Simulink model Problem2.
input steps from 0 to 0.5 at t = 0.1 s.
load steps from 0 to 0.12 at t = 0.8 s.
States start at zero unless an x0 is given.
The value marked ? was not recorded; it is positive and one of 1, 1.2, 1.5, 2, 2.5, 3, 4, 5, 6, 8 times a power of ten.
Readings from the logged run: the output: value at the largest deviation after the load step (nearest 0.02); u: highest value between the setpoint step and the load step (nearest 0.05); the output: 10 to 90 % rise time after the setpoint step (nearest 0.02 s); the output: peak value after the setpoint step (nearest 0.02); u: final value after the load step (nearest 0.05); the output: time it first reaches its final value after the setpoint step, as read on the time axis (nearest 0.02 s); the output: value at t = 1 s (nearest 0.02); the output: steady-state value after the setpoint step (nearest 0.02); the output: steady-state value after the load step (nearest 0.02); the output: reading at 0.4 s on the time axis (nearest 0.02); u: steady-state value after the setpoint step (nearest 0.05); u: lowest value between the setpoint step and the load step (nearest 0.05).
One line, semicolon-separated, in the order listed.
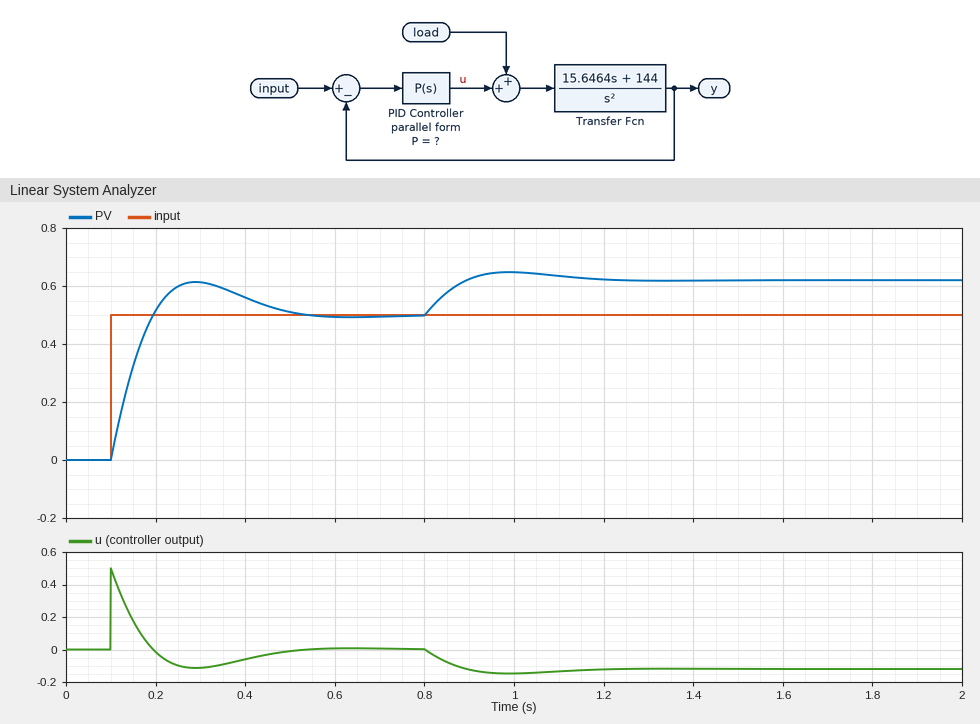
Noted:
0.64; 0.50; 0.08 s; 0.62; -0.10; 0.20 s; 0.64; 0.50; 0.62; 0.56; 0.00; -0.10
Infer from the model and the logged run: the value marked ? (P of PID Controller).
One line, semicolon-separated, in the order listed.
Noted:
1
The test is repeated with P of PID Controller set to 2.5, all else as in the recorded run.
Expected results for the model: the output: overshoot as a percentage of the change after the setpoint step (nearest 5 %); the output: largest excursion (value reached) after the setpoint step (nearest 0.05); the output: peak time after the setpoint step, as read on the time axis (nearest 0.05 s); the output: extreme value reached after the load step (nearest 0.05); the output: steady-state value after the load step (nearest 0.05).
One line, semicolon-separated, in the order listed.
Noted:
15 %; 0.55; 0.20 s; 0.55; 0.55
